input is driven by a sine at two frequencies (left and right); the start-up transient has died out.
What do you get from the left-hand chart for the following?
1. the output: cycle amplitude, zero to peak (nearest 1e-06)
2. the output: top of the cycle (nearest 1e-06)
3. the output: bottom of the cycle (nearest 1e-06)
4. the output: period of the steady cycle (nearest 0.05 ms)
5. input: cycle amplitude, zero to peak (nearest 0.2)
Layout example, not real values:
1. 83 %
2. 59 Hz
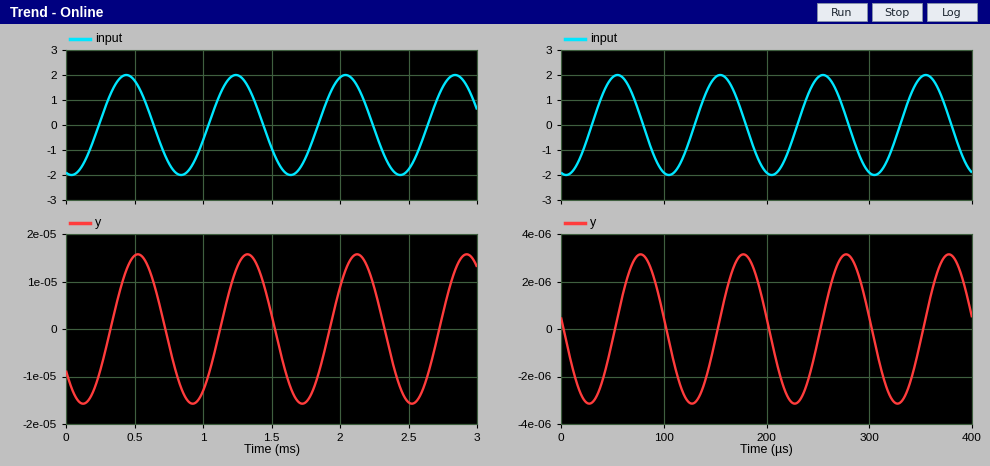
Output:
1. 0.000016
2. 0.000016
3. -0.000016
4. 0.80 ms
5. 2.0
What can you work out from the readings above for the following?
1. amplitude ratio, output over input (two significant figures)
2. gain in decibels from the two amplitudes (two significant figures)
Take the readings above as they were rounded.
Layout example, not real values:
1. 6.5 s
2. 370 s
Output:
1. 0.0000080
2. -100 dB
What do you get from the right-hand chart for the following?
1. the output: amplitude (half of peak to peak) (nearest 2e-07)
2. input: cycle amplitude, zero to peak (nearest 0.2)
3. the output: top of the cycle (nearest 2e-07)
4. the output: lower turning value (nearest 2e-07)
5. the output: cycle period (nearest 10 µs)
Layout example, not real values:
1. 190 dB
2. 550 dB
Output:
1. 0.0000032
2. 2.0
3. 0.0000032
4. -0.0000032
5. 100 µs
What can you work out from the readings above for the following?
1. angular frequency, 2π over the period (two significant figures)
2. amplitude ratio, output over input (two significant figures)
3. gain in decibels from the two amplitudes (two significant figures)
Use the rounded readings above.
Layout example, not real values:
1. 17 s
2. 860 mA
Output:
1. 0.063 rad/µs
2. 0.0000016
3. -120 dB
